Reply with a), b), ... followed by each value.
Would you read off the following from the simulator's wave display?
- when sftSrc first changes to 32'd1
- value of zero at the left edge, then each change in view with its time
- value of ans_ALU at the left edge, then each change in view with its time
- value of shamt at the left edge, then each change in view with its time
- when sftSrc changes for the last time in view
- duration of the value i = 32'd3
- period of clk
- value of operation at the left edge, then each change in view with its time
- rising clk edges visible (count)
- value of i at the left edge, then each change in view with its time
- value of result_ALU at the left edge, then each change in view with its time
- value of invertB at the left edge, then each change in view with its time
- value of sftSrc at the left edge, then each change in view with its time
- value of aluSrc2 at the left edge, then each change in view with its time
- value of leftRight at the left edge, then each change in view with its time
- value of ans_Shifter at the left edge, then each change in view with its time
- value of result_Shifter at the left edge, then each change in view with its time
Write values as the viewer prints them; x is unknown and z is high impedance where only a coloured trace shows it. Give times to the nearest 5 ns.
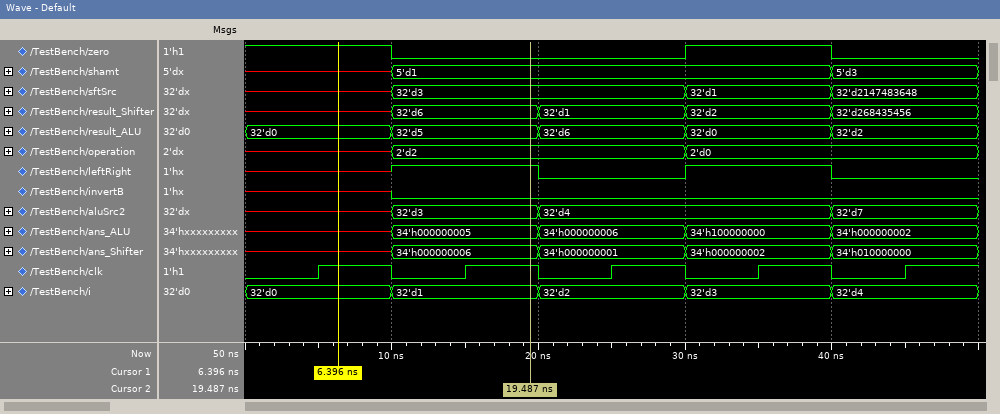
a) 30 ns
b) 1, 0 at 10 ns, 1 at 30 ns, 0 at 40 ns
c) x, 34'h000000005 at 10 ns, 34'h000000006 at 20 ns, 34'h100000000 at 30 ns, 34'h000000002 at 40 ns
d) x, 5'd1 at 10 ns, 5'd3 at 40 ns
e) 40 ns
f) 10 ns
g) 10 ns
h) x, 2'd2 at 10 ns, 2'd0 at 30 ns
i) 5
j) 32'd0, 32'd1 at 10 ns, 32'd2 at 20 ns, 32'd3 at 30 ns, 32'd4 at 40 ns
k) 32'd0, 32'd5 at 10 ns, 32'd6 at 20 ns, 32'd0 at 30 ns, 32'd2 at 40 ns
l) x, 0 at 10 ns
m) x, 32'd3 at 10 ns, 32'd1 at 30 ns, 32'd2147483648 at 40 ns
n) x, 32'd3 at 10 ns, 32'd4 at 20 ns, 32'd7 at 40 ns
o) x, 1 at 10 ns, 0 at 20 ns, 1 at 30 ns, 0 at 40 ns
p) x, 34'h000000006 at 10 ns, 34'h000000001 at 20 ns, 34'h000000002 at 30 ns, 34'h010000000 at 40 ns
q) x, 32'd6 at 10 ns, 32'd1 at 20 ns, 32'd2 at 30 ns, 32'd268435456 at 40 ns
